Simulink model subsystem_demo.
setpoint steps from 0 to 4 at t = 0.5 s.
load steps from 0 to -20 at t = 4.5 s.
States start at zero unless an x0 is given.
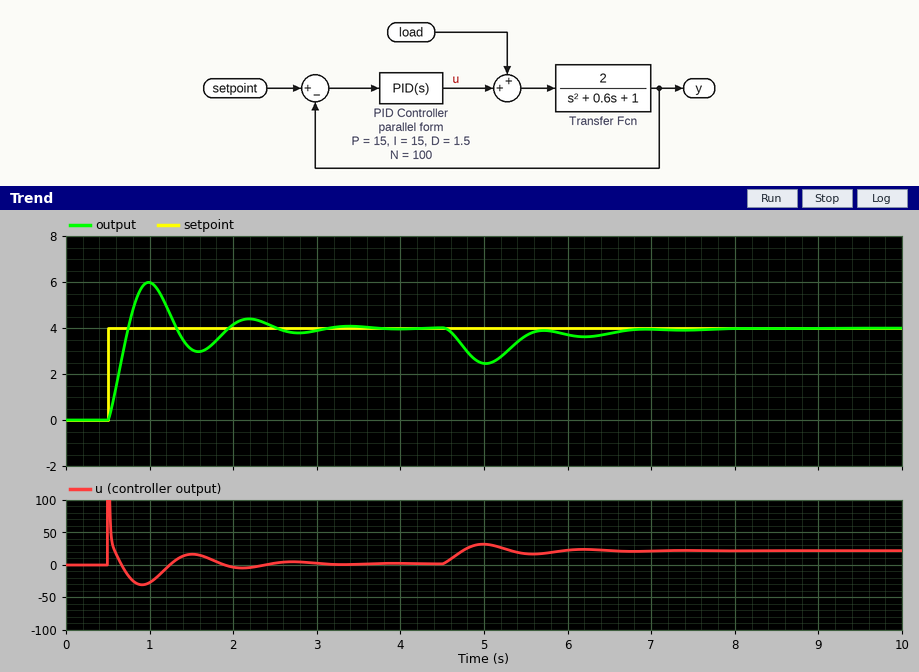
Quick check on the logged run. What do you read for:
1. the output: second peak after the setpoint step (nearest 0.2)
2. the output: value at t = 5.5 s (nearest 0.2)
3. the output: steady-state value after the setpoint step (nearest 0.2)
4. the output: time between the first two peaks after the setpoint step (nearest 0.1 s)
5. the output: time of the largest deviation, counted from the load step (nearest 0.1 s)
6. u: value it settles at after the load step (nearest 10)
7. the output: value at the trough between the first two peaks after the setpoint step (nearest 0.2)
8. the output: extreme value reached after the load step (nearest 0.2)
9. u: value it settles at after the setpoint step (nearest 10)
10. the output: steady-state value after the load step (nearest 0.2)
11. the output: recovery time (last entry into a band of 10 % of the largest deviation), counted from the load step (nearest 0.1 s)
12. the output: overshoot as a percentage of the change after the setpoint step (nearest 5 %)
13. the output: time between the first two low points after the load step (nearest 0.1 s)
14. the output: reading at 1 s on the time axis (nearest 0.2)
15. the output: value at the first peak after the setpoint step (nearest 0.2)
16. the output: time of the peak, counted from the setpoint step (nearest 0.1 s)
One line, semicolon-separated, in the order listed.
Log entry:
4.4; 3.6; 4.0; 1.2 s; 0.5 s; 20; 3.0; 2.4; 0; 4.0; 2.1 s; 50 %; 1.2 s; 6.0; 6.0; 0.5 s
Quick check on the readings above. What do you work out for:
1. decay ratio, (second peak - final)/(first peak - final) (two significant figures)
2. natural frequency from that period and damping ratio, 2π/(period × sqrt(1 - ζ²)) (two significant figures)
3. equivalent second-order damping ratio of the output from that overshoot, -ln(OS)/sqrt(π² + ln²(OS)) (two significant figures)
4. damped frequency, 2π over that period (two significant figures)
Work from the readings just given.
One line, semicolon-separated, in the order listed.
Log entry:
0.20; 5.4 rad/s; 0.22; 5.2 rad/s
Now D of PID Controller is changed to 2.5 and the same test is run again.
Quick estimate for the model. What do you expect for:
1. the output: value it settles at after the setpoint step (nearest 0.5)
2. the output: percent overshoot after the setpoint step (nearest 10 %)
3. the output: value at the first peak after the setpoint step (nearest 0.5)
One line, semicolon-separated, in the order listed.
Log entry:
4.0; 30 %; 5.5
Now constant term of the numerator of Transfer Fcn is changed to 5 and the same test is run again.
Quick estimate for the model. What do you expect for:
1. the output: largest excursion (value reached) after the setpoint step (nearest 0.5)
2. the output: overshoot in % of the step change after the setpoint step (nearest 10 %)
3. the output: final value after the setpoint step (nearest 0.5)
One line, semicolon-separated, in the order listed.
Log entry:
5.5; 40 %; 4.0
